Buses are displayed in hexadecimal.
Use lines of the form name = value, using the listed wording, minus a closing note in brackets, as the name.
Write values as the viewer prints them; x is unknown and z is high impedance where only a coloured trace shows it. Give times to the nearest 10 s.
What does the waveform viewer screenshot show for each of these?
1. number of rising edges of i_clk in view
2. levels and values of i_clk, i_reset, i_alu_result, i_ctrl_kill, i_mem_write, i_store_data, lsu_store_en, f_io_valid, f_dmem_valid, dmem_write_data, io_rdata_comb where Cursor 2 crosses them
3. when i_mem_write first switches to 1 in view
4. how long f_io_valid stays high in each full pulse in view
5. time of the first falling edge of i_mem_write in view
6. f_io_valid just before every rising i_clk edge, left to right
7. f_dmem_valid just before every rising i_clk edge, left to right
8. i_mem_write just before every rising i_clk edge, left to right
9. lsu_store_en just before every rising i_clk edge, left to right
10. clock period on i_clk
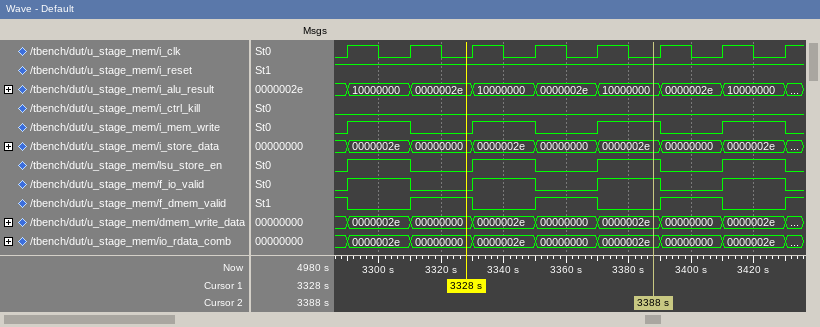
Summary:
number of rising edges of i_clk in view = 8
levels and values of i_clk, i_reset, i_alu_result, i_ctrl_kill, i_mem_write, i_store_data, lsu_store_en, f_io_valid, f_dmem_valid, dmem_write_data, io_rdata_comb where Cursor 2 crosses them = i_clk=0, i_reset=1, i_alu_result=10000000, i_ctrl_kill=0, i_mem_write=1, i_store_data=0000002e, lsu_store_en=1, f_io_valid=1, f_dmem_valid=0, dmem_write_data=0000002e, io_rdata_comb=0000002e
when i_mem_write first switches to 1 in view = 3290 s
how long f_io_valid stays high in each full pulse in view = 20 s, 20 s, 20 s, 20 s
time of the first falling edge of i_mem_write in view = 3310 s
f_io_valid just before every rising i_clk edge, left to right = 0 1 0 1 0 1 0 1
f_dmem_valid just before every rising i_clk edge, left to right = 1 0 1 0 1 0 1 0
i_mem_write just before every rising i_clk edge, left to right = 0 1 0 1 0 1 0 1
lsu_store_en just before every rising i_clk edge, left to right = 0 1 0 1 0 1 0 1
clock period on i_clk = 20 s
